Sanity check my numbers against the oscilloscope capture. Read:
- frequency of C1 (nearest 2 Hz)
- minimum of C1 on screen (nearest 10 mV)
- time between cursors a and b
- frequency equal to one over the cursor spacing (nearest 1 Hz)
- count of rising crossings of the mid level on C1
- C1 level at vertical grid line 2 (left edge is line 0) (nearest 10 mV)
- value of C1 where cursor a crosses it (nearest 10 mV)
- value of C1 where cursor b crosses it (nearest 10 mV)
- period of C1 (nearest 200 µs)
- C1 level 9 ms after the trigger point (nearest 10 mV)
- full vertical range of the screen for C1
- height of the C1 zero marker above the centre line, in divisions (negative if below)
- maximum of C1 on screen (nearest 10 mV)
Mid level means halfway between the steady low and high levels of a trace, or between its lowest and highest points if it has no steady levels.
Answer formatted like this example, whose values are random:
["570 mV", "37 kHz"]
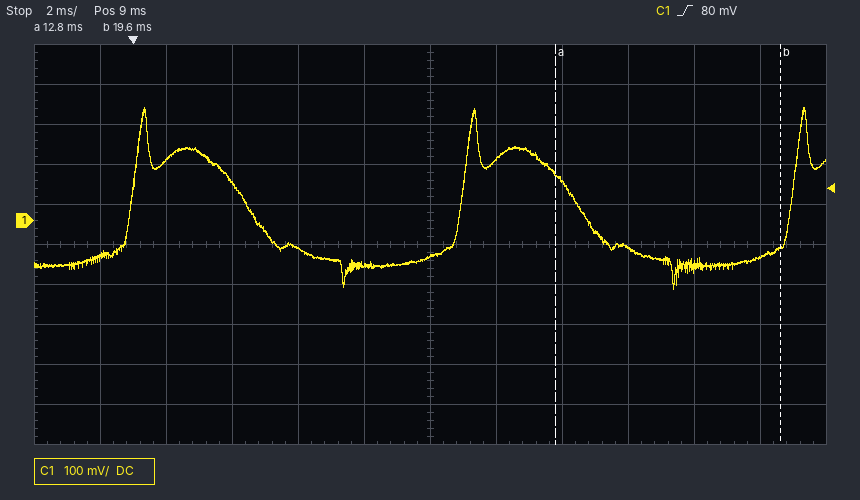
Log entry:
["100 Hz", "-170 mV", "6.8 ms", "147 Hz", "3", "150 mV", "120 mV", "-70 mV", "10.0 ms", "-90 mV", "1 V", "+0.6 div", "280 mV"]
